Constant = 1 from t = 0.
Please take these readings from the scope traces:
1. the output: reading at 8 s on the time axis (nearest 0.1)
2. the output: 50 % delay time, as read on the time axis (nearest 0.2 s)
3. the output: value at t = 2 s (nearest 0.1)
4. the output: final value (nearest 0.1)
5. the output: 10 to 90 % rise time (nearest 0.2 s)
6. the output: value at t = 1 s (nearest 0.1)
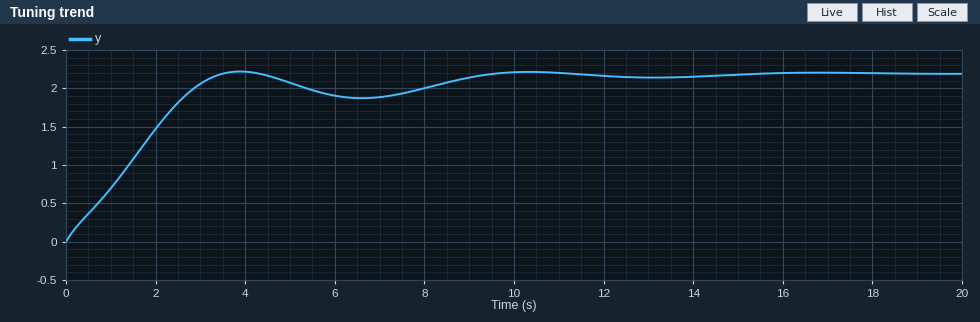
2.0
1.6 s
1.5
2.2
2.6 s
0.7
